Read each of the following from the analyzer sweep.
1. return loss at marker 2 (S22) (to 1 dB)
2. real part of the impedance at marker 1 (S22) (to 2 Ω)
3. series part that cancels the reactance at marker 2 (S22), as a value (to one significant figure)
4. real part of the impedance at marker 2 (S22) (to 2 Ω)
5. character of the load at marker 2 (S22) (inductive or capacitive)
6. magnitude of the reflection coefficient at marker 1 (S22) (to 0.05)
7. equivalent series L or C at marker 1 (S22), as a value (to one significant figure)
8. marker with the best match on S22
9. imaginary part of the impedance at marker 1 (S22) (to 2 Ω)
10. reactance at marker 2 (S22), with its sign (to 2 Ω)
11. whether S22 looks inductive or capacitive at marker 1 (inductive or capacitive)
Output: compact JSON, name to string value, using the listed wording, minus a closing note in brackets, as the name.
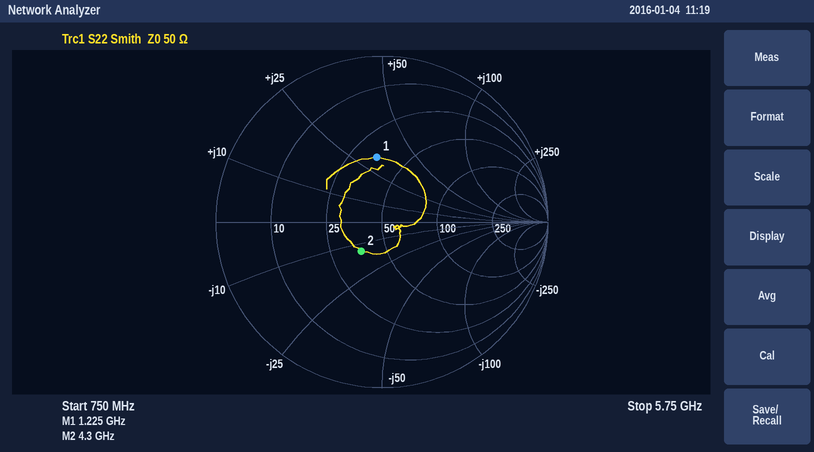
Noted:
{"return loss at marker 2 (S22)": "13 dB", "real part of the impedance at marker 1 (S22)": "34 Ω", "series part that cancels the reactance at marker 2 (S22), as a value": "500 pH", "real part of the impedance at marker 2 (S22)": "36 Ω", "character of the load at marker 2 (S22)": "capacitive", "magnitude of the reflection coefficient at marker 1 (S22)": "0.40", "equivalent series L or C at marker 1 (S22), as a value": "4 nH", "marker with the best match on S22": "marker 2", "imaginary part of the impedance at marker 1 (S22)": "+32 Ω", "reactance at marker 2 (S22), with its sign": "-14 Ω", "whether S22 looks inductive or capacitive at marker 1": "inductive"}
